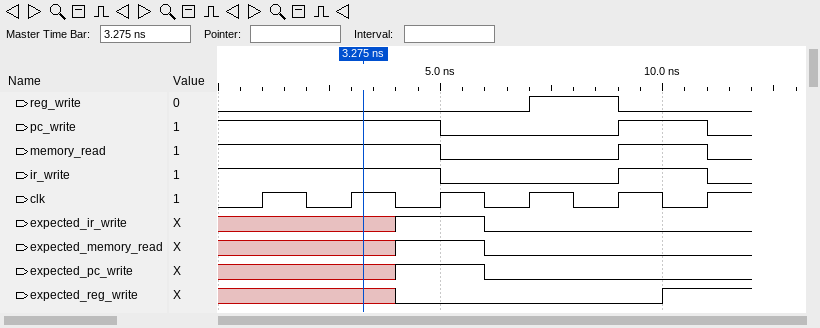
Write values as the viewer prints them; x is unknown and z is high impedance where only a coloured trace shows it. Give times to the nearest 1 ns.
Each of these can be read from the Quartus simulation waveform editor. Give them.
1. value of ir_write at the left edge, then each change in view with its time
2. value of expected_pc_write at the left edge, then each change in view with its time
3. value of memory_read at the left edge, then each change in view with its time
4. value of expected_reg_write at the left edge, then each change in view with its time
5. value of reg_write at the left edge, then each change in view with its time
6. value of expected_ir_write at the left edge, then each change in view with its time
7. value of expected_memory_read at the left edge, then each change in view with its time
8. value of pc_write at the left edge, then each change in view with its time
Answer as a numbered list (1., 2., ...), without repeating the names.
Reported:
1. 1, 0 at 5 ns, 1 at 9 ns, 0 at 11 ns
2. x, 1 at 4 ns, 0 at 6 ns
3. 1, 0 at 5 ns, 1 at 9 ns, 0 at 11 ns
4. x, 0 at 4 ns, 1 at 10 ns
5. 0, 1 at 7 ns, 0 at 9 ns
6. x, 1 at 4 ns, 0 at 6 ns
7. x, 1 at 4 ns, 0 at 6 ns
8. 1, 0 at 5 ns, 1 at 9 ns, 0 at 11 ns
